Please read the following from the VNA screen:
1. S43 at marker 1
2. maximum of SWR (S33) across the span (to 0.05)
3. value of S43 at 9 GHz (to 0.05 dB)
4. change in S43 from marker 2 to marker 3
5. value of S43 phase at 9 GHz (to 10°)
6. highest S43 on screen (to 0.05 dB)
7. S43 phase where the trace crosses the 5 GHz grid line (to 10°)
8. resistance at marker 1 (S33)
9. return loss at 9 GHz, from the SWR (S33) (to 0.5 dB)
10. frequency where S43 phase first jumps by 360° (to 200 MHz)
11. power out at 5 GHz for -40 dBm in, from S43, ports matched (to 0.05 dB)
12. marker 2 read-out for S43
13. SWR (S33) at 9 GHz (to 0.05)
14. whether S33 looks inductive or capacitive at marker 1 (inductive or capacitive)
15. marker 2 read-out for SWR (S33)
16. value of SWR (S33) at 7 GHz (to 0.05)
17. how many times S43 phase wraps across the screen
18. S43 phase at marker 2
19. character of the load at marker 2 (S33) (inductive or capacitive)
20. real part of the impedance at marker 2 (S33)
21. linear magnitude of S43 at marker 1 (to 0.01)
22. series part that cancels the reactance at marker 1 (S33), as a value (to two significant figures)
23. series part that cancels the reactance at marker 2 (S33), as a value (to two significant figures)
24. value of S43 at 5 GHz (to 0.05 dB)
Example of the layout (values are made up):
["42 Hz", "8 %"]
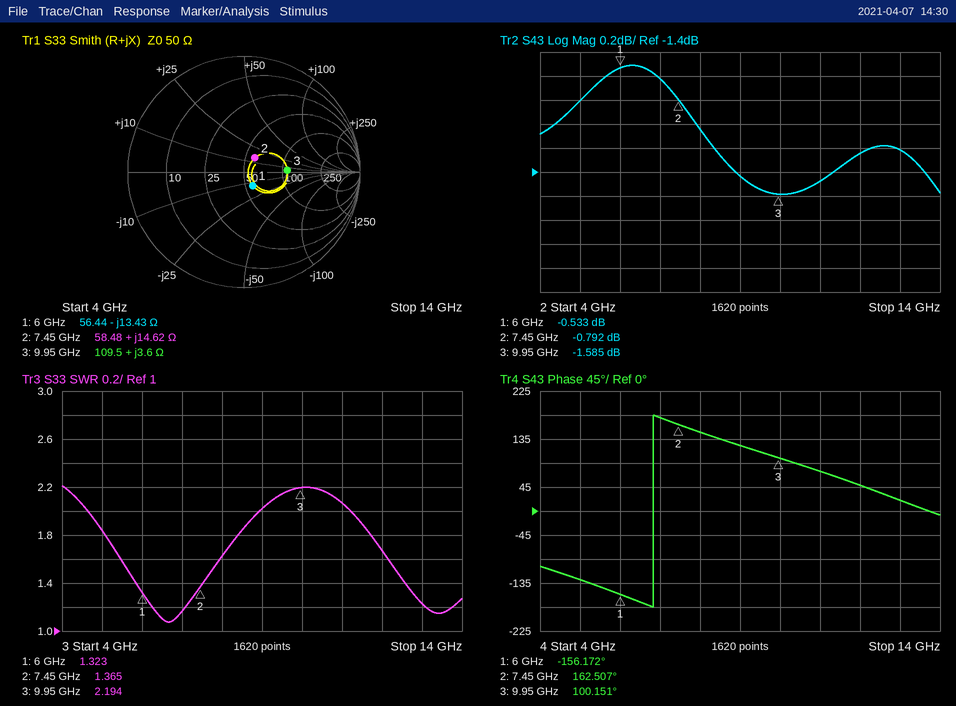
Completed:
["-0.533 dB", "2.20", "-1.45 dB", "-0.793 dB", "120°", "-0.50 dB", "-130°", "56.44 Ω", "9.5 dB", "6.8 GHz", "-40.80 dBm", "-0.792 dB", "2.00", "capacitive", "1.365", "1.15", "1", "162.507°", "inductive", "58.48 Ω", "0.94", "360 pH", "1.5 pF", "-0.80 dB"]
